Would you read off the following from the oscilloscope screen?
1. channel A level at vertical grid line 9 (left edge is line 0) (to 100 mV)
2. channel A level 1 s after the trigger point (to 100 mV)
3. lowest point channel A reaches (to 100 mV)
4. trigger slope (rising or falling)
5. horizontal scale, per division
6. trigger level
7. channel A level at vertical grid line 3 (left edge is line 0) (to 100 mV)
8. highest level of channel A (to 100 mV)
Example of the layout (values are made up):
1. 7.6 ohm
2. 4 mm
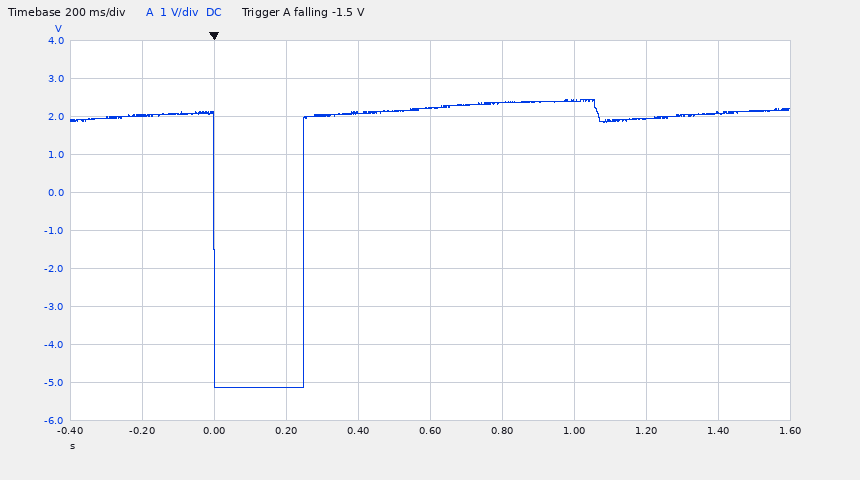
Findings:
1. 2.1 V
2. 2.4 V
3. -5.1 V
4. falling
5. 200 ms
6. -1.5 V
7. -5.1 V
8. 2.4 V
